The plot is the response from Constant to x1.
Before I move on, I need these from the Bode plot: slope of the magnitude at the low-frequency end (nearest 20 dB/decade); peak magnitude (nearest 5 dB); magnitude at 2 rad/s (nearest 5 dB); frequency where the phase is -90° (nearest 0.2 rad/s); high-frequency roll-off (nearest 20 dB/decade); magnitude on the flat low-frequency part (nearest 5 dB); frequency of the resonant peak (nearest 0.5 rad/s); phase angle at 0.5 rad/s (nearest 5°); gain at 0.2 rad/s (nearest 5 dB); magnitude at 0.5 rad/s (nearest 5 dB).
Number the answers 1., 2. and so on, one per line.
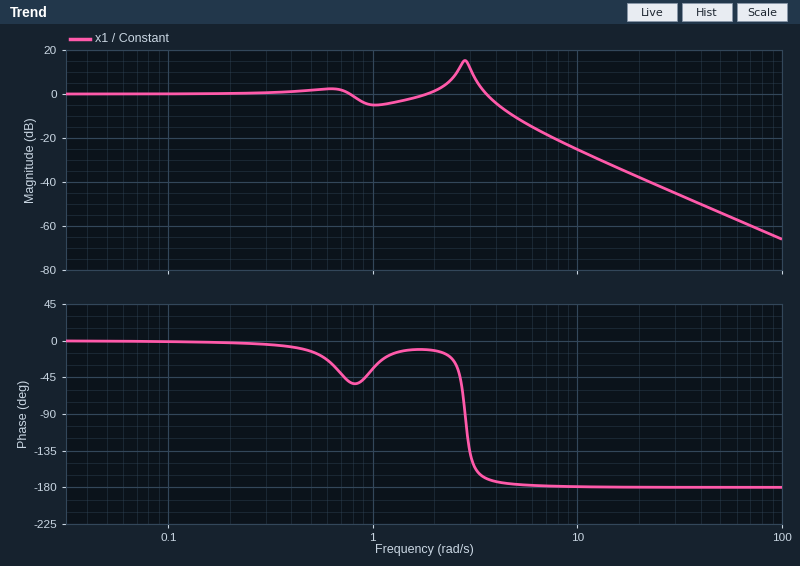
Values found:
1. 0 dB/decade
2. 15 dB
3. 0 dB
4. 2.8 rad/s
5. -40 dB/decade
6. 0 dB
7. 3.0 rad/s
8. -15°
9. 0 dB
10. 0 dB
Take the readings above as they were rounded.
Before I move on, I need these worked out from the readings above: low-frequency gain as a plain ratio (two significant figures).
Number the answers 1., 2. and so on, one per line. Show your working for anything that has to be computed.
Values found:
1. 10^(0 / 20) = 1.0
